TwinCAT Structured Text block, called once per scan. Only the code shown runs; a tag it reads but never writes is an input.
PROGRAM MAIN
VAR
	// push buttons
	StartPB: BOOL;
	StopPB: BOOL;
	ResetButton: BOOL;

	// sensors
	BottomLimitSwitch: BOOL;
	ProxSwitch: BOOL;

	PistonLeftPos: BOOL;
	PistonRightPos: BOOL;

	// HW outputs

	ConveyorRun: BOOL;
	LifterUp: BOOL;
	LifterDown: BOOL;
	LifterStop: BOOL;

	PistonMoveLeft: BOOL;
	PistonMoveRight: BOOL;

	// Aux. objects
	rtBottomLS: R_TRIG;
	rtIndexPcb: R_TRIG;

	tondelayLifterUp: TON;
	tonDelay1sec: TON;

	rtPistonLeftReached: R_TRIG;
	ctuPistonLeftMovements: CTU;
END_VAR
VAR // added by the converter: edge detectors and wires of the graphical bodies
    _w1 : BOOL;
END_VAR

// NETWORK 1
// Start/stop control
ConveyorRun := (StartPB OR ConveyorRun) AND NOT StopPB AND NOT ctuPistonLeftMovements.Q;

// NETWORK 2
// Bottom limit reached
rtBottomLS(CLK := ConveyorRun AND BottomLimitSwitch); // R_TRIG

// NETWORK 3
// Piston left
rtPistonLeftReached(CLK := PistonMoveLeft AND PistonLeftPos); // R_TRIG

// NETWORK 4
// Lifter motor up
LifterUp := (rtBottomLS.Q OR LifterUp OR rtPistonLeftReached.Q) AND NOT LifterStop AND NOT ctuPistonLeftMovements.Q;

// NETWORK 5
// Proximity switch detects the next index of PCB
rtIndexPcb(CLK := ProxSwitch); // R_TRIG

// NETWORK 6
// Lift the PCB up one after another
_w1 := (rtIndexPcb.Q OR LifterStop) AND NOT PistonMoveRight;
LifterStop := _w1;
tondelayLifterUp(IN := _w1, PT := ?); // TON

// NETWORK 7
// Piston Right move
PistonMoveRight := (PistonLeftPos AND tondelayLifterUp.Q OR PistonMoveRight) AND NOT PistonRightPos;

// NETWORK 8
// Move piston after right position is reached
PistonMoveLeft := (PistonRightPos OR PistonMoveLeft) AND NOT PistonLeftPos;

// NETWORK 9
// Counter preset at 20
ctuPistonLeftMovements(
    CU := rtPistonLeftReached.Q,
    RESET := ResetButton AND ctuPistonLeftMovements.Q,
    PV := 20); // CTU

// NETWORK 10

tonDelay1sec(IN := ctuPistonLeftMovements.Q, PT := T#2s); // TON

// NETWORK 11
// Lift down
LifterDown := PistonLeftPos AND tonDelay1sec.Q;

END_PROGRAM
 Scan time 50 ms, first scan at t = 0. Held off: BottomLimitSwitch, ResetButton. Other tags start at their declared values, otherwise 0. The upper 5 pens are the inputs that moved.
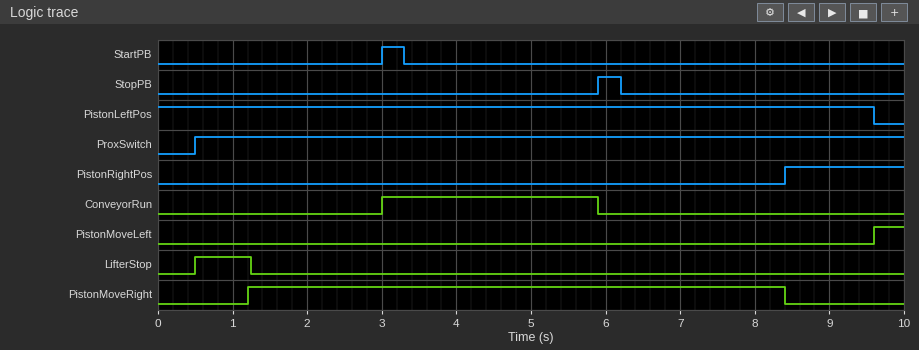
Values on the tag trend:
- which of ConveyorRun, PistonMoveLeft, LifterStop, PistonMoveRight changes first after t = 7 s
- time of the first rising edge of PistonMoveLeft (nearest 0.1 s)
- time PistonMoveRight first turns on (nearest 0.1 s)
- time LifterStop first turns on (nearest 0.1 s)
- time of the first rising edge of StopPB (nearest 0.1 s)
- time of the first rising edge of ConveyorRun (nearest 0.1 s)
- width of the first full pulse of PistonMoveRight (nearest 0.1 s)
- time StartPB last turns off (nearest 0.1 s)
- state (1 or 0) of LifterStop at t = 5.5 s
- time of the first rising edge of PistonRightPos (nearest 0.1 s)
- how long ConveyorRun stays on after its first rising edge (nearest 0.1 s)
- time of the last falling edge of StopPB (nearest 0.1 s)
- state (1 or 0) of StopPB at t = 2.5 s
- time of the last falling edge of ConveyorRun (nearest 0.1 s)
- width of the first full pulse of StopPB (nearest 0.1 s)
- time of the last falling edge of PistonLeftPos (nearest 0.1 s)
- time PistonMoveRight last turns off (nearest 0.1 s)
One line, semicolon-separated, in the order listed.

PistonMoveRight; 9.6 s; 1.2 s; 0.5 s; 5.9 s; 3.0 s; 7.2 s; 3.3 s; 0; 8.4 s; 2.9 s; 6.2 s; 0; 5.9 s; 0.3 s; 9.6 s; 8.4 s
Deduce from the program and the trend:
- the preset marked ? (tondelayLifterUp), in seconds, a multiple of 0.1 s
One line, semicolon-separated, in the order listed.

0.7 s
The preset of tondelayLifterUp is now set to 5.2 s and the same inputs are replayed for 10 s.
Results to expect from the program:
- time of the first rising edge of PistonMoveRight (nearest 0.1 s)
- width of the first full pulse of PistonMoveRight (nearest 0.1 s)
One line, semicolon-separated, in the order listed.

5.7 s; 2.7 s
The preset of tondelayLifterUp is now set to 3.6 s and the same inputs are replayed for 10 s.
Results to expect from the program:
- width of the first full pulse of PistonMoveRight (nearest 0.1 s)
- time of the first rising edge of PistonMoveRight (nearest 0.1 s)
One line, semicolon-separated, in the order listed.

4.3 s; 4.1 s
